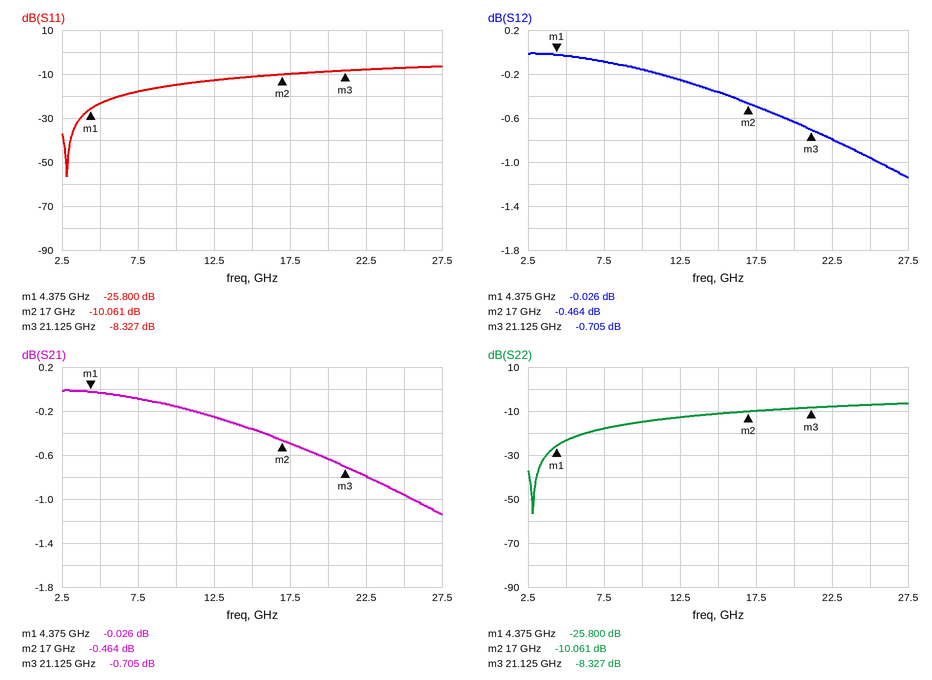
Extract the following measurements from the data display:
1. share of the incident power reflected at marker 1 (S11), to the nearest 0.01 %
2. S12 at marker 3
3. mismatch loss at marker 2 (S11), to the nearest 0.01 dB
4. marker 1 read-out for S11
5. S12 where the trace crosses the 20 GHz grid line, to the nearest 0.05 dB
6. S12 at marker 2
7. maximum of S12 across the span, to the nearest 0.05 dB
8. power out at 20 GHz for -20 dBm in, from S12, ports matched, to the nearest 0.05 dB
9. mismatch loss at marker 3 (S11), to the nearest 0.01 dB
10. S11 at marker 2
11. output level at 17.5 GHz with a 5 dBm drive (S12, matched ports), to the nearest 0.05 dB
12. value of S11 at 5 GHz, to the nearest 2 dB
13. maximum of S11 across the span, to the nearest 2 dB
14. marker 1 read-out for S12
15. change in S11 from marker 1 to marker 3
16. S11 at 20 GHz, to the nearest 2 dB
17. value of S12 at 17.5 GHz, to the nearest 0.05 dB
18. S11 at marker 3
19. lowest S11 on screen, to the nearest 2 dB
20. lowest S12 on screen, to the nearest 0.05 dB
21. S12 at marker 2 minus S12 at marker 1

0.26 %
-0.705 dB
0.45 dB
-25.800 dB
-0.65 dB
-0.464 dB
0.00 dB
-20.65 dBm
0.69 dB
-10.061 dB
4.50 dBm
-24 dB
-6 dB
-0.026 dB
17.473 dB
-8 dB
-0.50 dB
-8.327 dB
-56 dB
-1.15 dB
-0.438 dB
